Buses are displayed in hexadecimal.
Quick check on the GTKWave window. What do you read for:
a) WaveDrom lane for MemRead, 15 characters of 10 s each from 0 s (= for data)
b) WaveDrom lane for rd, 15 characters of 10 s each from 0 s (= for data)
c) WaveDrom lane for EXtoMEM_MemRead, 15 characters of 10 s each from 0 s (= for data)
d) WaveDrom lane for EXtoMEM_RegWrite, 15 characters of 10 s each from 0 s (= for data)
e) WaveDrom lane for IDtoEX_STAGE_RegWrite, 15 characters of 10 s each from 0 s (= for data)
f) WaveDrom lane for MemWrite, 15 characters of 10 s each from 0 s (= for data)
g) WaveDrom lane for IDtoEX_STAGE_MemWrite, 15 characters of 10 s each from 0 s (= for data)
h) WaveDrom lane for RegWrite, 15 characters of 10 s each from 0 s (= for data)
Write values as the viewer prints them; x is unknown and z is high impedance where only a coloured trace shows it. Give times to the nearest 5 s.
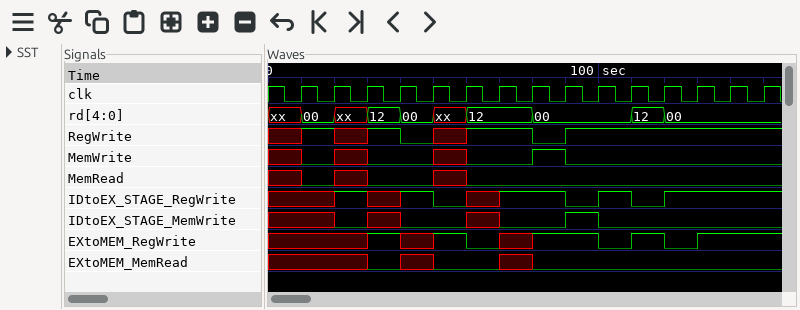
{name: 'MemRead', wave: 'x0x0.x0........'}
{name: 'rd', wave: 'x=x==x=.=..==..', data: '00 12 00 12 00 12 00'}
{name: 'EXtoMEM_MemRead', wave: 'x..0x0.x0......'}
{name: 'EXtoMEM_RegWrite', wave: 'x..1x10x1.0101.'}
{name: 'IDtoEX_STAGE_RegWrite', wave: 'x.1x10x1.0101..'}
{name: 'MemWrite', wave: 'x0x0.x0.10.....'}
{name: 'IDtoEX_STAGE_MemWrite', wave: 'x.0x0.x0.10....'}
{name: 'RegWrite', wave: 'x1x10x1.01.....'}
